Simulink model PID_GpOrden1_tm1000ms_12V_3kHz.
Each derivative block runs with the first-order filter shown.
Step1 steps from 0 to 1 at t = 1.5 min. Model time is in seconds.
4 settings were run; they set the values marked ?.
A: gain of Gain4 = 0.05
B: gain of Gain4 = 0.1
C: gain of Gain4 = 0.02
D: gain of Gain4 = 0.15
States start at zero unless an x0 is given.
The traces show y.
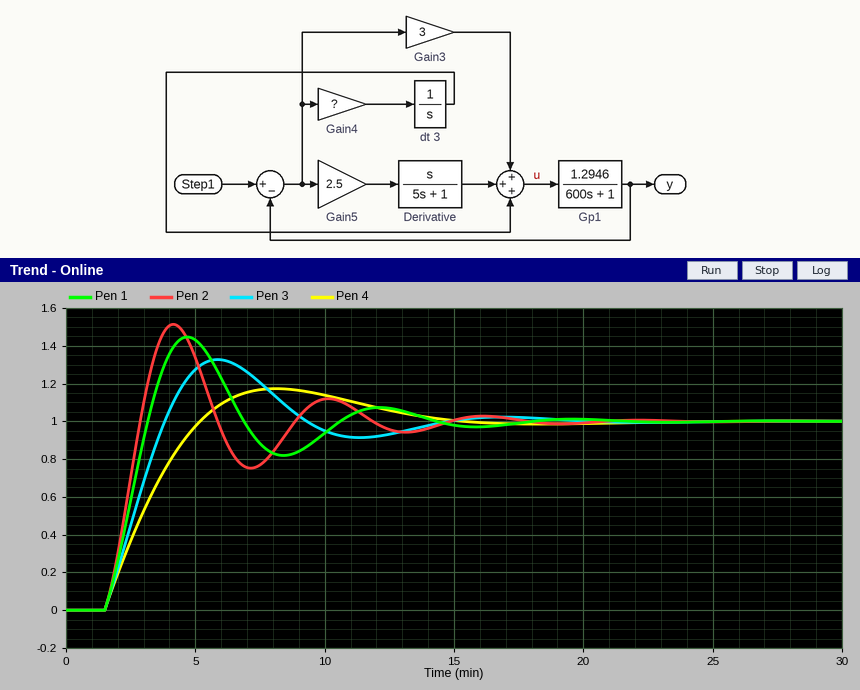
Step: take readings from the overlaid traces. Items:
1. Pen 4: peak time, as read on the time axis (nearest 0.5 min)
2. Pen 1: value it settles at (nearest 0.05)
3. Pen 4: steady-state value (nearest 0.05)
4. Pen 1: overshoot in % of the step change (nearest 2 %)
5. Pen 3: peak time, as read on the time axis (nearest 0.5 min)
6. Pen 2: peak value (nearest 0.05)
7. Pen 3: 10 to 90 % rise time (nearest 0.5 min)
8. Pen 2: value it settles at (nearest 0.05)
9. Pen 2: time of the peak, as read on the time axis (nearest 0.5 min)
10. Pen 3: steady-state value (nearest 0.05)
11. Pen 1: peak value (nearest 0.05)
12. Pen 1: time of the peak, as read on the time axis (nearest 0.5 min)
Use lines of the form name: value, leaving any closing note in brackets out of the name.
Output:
Pen 4: peak time, as read on the time axis: 8.0 min
Pen 1: value it settles at: 1.00
Pen 4: steady-state value: 1.00
Pen 1: overshoot in % of the step change: 44 %
Pen 3: peak time, as read on the time axis: 6.0 min
Pen 2: peak value: 1.50
Pen 3: 10 to 90 % rise time: 2.0 min
Pen 2: value it settles at: 1.00
Pen 2: time of the peak, as read on the time axis: 4.0 min
Pen 3: steady-state value: 1.00
Pen 1: peak value: 1.45
Pen 1: time of the peak, as read on the time axis: 4.5 min
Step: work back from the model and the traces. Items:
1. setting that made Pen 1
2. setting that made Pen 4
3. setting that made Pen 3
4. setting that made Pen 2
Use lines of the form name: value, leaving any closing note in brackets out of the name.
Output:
setting that made Pen 1: B
setting that made Pen 4: C
setting that made Pen 3: A
setting that made Pen 2: D
